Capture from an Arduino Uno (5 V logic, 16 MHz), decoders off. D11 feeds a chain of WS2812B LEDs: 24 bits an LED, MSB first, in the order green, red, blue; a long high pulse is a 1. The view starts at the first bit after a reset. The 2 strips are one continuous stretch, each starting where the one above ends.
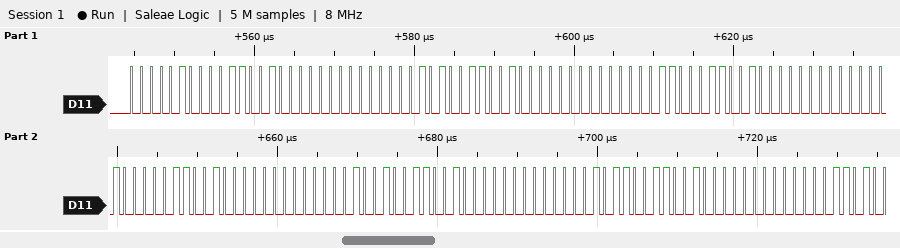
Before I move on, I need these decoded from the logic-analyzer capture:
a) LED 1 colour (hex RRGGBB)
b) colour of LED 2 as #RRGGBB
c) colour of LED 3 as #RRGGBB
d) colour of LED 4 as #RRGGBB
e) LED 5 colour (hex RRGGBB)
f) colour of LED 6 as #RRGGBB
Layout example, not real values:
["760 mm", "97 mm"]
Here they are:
["#320400", "#320500", "#320600", "#320800", "#320900", "#320B00"]
